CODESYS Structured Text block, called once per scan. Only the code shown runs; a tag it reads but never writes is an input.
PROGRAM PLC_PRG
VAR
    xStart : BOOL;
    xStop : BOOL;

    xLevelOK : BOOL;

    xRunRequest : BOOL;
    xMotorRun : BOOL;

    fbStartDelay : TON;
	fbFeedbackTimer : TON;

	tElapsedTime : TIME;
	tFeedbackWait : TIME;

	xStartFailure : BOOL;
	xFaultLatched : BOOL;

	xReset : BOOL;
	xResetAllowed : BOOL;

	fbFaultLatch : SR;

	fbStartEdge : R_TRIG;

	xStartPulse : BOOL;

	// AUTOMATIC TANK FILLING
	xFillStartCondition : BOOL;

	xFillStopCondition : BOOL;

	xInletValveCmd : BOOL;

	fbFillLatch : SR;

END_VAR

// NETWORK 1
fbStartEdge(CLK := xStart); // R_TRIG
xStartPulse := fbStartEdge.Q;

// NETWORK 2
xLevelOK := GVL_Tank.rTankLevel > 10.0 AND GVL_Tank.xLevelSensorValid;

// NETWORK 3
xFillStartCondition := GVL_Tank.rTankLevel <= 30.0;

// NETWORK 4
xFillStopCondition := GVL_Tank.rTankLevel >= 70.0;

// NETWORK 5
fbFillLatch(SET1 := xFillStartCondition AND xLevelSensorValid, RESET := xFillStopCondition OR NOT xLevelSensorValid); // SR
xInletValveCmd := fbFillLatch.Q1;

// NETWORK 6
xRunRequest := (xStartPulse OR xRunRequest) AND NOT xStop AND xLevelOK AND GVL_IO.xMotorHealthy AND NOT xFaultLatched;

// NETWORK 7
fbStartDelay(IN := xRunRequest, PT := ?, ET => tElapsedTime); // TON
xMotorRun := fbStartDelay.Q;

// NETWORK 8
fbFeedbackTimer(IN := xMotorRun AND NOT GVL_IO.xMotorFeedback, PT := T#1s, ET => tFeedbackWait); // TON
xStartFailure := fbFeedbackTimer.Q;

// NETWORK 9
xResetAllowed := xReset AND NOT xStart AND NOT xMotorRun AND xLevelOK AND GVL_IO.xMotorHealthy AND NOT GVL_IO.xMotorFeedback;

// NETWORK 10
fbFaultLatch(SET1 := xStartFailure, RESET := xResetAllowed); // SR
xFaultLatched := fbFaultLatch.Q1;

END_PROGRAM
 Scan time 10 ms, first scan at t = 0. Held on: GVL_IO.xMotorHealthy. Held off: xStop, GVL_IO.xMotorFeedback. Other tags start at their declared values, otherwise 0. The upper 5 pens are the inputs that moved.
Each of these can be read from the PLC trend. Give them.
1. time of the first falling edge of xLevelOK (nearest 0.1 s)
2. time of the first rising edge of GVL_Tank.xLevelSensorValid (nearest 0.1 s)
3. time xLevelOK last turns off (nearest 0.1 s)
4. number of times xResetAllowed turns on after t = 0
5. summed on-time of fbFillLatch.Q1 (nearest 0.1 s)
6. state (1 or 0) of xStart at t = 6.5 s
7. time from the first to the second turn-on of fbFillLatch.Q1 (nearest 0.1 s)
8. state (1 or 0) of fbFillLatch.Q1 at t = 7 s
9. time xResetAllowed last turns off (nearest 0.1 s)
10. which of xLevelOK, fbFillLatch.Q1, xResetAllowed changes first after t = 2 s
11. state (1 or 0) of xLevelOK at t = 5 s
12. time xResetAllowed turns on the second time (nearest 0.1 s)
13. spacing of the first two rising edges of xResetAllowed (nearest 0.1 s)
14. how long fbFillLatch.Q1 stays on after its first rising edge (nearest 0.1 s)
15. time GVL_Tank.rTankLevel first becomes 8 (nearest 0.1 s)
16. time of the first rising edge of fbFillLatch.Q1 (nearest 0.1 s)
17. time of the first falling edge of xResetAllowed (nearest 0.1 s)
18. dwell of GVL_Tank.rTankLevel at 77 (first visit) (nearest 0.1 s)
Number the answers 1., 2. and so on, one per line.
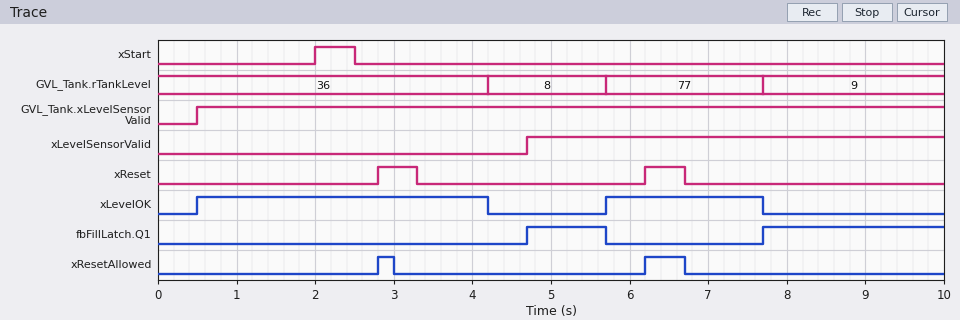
1. 4.2 s
2. 0.5 s
3. 7.7 s
4. 2
5. 3.3 s
6. 0
7. 3.0 s
8. 0
9. 6.7 s
10. xResetAllowed
11. 0
12. 6.2 s
13. 3.4 s
14. 1.0 s
15. 4.2 s
16. 4.7 s
17. 3.0 s
18. 2.0 s
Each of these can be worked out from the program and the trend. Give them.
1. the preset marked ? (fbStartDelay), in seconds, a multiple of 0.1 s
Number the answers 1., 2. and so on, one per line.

1. 1.0 s
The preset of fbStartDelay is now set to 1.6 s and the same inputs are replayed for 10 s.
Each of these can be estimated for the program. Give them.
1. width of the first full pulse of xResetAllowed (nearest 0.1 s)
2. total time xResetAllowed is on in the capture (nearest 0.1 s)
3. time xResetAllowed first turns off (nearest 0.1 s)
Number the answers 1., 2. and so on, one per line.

1. 0.5 s
2. 1.0 s
3. 3.3 s
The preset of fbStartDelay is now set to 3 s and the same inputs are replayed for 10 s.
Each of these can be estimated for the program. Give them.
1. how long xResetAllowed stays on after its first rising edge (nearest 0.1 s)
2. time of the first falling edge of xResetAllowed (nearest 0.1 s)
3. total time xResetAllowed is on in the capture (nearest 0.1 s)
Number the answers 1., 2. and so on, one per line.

1. 0.5 s
2. 3.3 s
3. 1.0 s
